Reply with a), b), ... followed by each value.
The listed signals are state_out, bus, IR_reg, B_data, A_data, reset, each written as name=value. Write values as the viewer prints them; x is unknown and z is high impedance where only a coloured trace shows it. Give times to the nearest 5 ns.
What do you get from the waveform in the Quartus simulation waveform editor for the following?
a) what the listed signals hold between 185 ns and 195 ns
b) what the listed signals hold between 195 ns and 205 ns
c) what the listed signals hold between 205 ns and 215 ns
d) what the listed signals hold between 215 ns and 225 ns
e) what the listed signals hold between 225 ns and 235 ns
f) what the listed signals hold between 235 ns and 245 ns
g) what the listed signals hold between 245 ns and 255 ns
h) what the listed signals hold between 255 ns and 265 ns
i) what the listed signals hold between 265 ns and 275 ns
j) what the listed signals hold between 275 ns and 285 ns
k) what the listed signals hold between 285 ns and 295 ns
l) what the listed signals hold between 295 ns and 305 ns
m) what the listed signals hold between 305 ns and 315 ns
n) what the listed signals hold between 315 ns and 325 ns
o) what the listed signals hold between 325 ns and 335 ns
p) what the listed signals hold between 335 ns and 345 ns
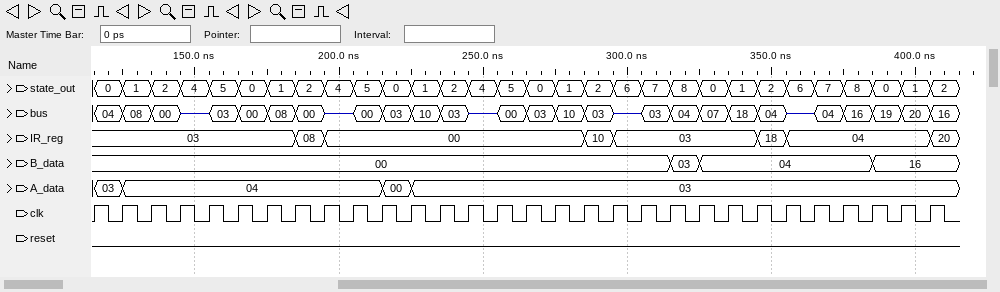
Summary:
a) state_out=2, bus=00, IR_reg=08, B_data=00, A_data=04, reset=0
b) state_out=4, bus=z, IR_reg=00, B_data=00, A_data=04, reset=0
c) state_out=5, bus=00, IR_reg=00, B_data=00, A_data=04, reset=0
d) state_out=0, bus=03, IR_reg=00, B_data=00, A_data=00, reset=0
e) state_out=1, bus=10, IR_reg=00, B_data=00, A_data=03, reset=0
f) state_out=2, bus=03, IR_reg=00, B_data=00, A_data=03, reset=0
g) state_out=4, bus=z, IR_reg=00, B_data=00, A_data=03, reset=0
h) state_out=5, bus=00, IR_reg=00, B_data=00, A_data=03, reset=0
i) state_out=0, bus=03, IR_reg=00, B_data=00, A_data=03, reset=0
j) state_out=1, bus=10, IR_reg=00, B_data=00, A_data=03, reset=0
k) state_out=2, bus=03, IR_reg=10, B_data=00, A_data=03, reset=0
l) state_out=6, bus=z, IR_reg=03, B_data=00, A_data=03, reset=0
m) state_out=7, bus=03, IR_reg=03, B_data=00, A_data=03, reset=0
n) state_out=8, bus=04, IR_reg=03, B_data=03, A_data=03, reset=0
o) state_out=0, bus=07, IR_reg=03, B_data=04, A_data=03, reset=0
p) state_out=1, bus=18, IR_reg=03, B_data=04, A_data=03, reset=0
